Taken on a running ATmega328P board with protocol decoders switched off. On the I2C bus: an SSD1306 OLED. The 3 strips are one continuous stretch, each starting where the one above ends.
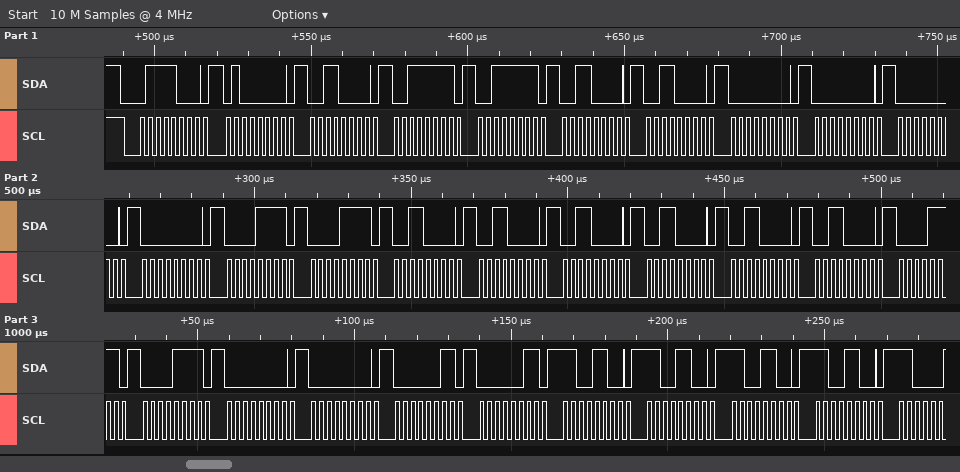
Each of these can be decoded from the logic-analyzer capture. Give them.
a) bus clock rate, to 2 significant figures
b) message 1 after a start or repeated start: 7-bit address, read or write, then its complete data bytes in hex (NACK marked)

400 kHz
0x3C write: 40 30 3F 3F 30 30 00 00 00 00 0F 0F 30 30 30 30 30 30 0F 0F 00 00 03 03 CC CC CC CC
